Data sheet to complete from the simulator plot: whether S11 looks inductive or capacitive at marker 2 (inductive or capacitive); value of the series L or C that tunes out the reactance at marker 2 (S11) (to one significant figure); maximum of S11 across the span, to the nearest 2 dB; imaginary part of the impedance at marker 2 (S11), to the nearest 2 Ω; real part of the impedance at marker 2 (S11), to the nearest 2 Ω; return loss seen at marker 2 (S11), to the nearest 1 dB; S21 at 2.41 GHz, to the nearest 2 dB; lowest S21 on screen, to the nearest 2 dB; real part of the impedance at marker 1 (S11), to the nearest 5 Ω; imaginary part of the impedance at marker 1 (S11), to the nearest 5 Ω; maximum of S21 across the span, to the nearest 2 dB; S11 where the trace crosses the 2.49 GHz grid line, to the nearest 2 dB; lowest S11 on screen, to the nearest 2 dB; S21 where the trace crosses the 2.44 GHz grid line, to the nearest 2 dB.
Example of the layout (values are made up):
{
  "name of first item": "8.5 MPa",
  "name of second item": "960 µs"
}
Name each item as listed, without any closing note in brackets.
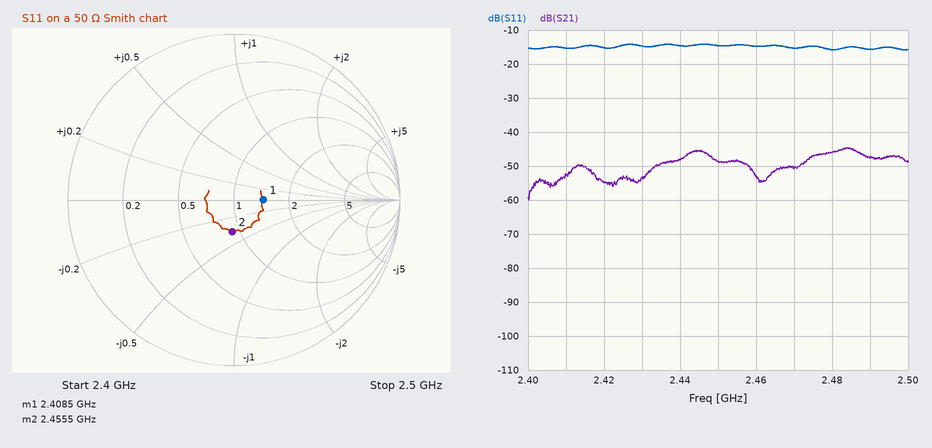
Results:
{
  "whether S11 looks inductive or capacitive at marker 2": "capacitive",
  "value of the series L or C that tunes out the reactance at marker 2 (S11)": "1 nH",
  "maximum of S11 across the span, to the nearest 2 dB": "-14 dB",
  "imaginary part of the impedance at marker 2 (S11), to the nearest 2 Ω": "-18 Ω",
  "real part of the impedance at marker 2 (S11), to the nearest 2 Ω": "46 Ω",
  "return loss seen at marker 2 (S11), to the nearest 1 dB": "14 dB",
  "S21 at 2.41 GHz, to the nearest 2 dB": "-52 dB",
  "lowest S21 on screen, to the nearest 2 dB": "-60 dB",
  "real part of the impedance at marker 1 (S11), to the nearest 5 Ω": "70 Ω",
  "imaginary part of the impedance at marker 1 (S11), to the nearest 5 Ω": "0 Ω",
  "maximum of S21 across the span, to the nearest 2 dB": "-44 dB",
  "S11 where the trace crosses the 2.49 GHz grid line, to the nearest 2 dB": "-16 dB",
  "lowest S11 on screen, to the nearest 2 dB": "-16 dB",
  "S21 where the trace crosses the 2.44 GHz grid line, to the nearest 2 dB": "-48 dB"
}
